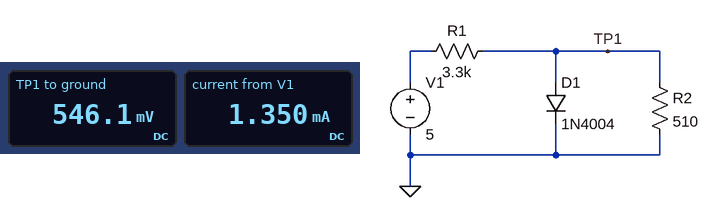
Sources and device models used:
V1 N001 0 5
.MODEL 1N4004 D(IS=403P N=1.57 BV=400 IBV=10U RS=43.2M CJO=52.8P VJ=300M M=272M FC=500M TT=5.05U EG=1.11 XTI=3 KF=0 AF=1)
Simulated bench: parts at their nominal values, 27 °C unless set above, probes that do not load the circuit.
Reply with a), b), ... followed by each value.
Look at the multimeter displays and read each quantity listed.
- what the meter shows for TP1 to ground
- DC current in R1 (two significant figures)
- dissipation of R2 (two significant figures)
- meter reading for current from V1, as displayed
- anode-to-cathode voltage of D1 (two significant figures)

a) 546.1 mV
b) 1.3 mA
c) 580 µW
d) 1.350 mA
e) 550 mV
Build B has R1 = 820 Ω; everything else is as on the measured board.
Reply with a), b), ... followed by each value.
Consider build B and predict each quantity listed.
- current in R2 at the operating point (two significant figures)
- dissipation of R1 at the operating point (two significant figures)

a) 1.3 mA
b) 23 mW
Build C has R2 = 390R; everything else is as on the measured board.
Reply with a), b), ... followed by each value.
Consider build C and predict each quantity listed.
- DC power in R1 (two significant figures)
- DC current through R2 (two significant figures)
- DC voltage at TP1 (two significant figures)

a) 6.1 mW
b) 1.3 mA
c) 500 mV
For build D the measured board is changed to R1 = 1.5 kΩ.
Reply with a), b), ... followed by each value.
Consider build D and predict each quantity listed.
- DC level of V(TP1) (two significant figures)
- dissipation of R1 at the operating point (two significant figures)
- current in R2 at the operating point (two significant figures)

a) 620 mV
b) 13 mW
c) 1.2 mA
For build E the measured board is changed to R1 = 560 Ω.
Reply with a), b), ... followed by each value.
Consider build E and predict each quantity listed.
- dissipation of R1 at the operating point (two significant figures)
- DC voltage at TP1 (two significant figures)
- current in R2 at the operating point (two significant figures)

a) 33 mW
b) 670 mV
c) 1.3 mA
